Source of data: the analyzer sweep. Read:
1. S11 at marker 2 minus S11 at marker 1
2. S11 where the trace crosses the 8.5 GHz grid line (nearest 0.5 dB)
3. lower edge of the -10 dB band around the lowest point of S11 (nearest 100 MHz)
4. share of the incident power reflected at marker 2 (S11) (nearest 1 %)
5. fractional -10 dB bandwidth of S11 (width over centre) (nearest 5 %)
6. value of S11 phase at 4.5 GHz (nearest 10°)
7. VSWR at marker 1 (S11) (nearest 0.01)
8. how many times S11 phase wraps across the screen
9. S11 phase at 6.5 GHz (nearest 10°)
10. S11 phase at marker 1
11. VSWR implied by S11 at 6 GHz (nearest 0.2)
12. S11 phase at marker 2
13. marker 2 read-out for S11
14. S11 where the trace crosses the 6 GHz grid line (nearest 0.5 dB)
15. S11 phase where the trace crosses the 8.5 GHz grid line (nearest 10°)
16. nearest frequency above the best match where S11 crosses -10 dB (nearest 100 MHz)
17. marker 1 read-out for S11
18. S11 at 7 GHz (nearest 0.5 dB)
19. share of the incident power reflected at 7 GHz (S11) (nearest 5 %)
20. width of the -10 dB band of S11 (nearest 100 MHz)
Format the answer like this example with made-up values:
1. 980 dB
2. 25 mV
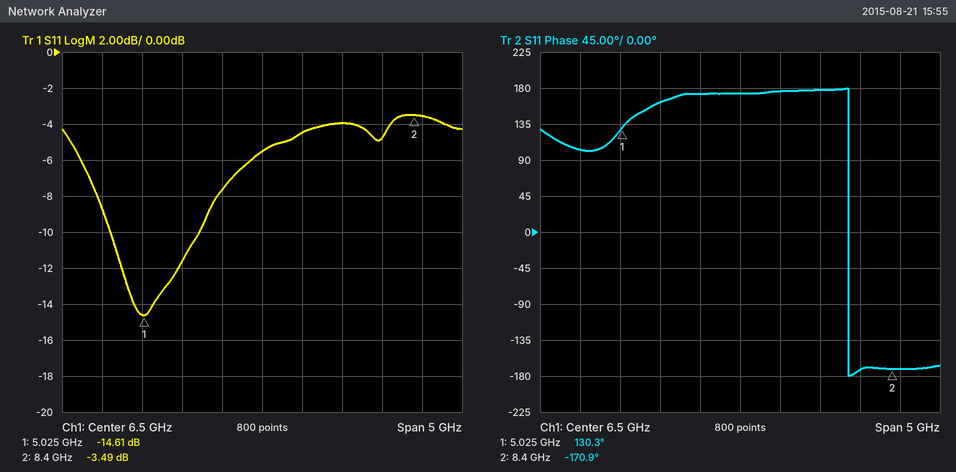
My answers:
1. 11.12 dB
2. -3.5 dB
3. 4.6 GHz
4. 45 %
5. 20 %
6. 100°
7. 1.46
8. 1
9. 170°
10. 130.3°
11. 2.4
12. -170.9°
13. -3.49 dB
14. -7.5 dB
15. -170°
16. 5.7 GHz
17. -14.61 dB
18. -4.5 dB
19. 35 %
20. 1.1 GHz
